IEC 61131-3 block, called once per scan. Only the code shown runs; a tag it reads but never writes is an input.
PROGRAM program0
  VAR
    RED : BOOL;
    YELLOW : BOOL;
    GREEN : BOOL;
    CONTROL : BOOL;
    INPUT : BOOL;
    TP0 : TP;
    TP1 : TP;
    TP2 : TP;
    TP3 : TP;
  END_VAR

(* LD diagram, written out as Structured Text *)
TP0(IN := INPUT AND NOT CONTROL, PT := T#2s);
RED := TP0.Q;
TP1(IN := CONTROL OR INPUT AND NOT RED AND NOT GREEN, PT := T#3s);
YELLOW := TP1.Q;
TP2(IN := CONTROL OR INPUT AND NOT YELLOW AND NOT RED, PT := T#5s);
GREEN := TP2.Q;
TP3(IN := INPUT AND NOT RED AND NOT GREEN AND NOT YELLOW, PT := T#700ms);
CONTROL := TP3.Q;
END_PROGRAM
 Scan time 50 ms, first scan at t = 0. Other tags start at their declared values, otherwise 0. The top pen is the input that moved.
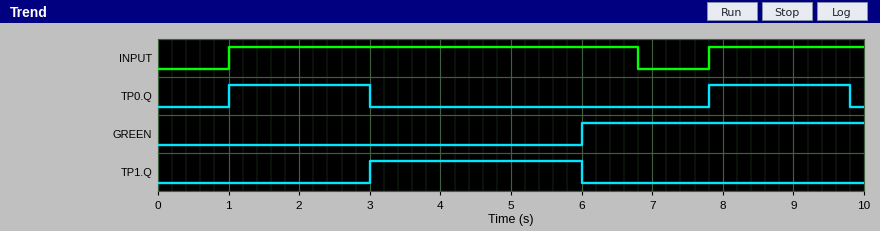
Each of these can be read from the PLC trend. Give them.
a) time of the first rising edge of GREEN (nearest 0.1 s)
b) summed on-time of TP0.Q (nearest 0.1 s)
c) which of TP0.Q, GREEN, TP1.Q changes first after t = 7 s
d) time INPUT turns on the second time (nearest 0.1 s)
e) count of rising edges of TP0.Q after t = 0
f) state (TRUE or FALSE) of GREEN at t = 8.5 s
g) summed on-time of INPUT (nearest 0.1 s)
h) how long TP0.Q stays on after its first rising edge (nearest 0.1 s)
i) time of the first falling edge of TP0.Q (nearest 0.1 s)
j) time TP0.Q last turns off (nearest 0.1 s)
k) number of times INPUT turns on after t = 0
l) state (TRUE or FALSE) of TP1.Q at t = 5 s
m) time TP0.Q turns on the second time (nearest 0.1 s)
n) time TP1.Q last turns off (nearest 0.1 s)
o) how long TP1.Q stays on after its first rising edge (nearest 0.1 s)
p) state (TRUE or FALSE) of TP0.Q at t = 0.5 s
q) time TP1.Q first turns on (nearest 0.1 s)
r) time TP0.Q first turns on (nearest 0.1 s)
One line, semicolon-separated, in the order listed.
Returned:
6.0 s; 4.0 s; TP0.Q; 7.8 s; 2; TRUE; 8.0 s; 2.0 s; 3.0 s; 9.8 s; 2; TRUE; 7.8 s; 6.0 s; 3.0 s; FALSE; 3.0 s; 1.0 s
